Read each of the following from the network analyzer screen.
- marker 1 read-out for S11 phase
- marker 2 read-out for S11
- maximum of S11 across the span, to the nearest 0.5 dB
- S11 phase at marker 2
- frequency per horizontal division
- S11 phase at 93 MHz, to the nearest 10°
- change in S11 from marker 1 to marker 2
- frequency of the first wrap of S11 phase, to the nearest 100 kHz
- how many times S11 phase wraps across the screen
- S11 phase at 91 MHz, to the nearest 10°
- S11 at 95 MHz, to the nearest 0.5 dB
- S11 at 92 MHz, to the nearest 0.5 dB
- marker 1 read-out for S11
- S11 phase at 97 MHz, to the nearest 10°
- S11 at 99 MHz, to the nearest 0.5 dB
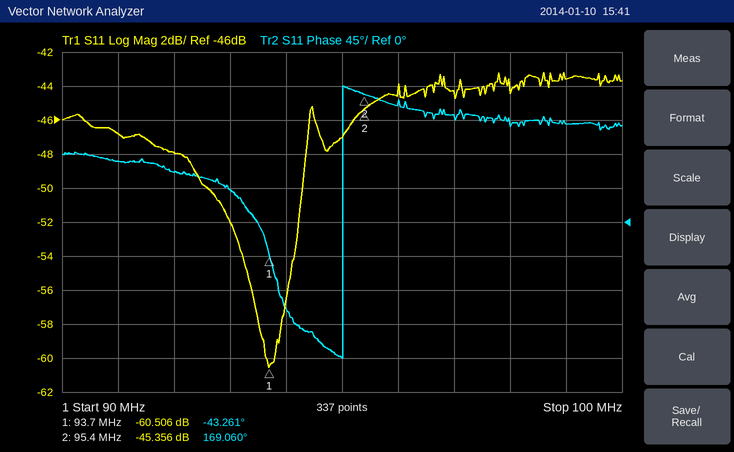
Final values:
-43.261°
-45.356 dB
-43.0 dB
169.060°
1 MHz
40°
15.150 dB
95.0 MHz
1
80°
-47.0 dB
-48.0 dB
-60.506 dB
140°
-43.5 dB
